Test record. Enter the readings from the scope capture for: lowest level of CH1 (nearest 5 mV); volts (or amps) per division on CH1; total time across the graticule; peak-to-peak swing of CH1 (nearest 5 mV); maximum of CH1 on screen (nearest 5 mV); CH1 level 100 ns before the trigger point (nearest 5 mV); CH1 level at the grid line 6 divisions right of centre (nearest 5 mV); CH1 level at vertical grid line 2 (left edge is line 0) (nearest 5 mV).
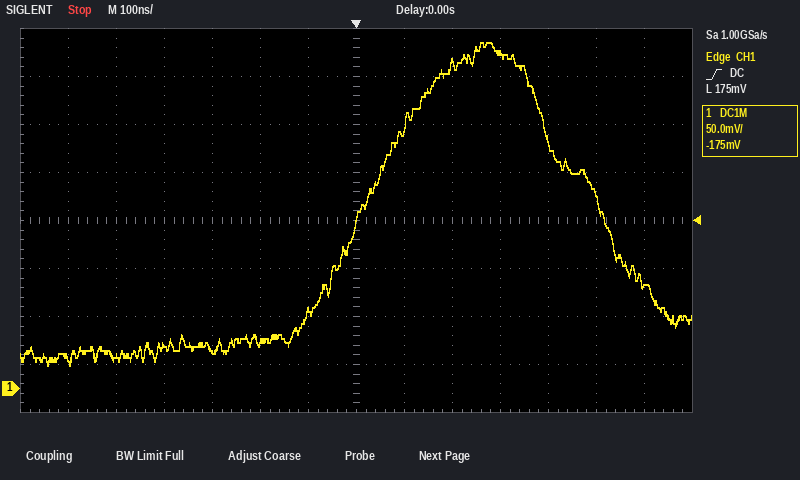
25 mV
50 mV
1.4 µs
335 mV
360 mV
80 mV
105 mV
35 mV
